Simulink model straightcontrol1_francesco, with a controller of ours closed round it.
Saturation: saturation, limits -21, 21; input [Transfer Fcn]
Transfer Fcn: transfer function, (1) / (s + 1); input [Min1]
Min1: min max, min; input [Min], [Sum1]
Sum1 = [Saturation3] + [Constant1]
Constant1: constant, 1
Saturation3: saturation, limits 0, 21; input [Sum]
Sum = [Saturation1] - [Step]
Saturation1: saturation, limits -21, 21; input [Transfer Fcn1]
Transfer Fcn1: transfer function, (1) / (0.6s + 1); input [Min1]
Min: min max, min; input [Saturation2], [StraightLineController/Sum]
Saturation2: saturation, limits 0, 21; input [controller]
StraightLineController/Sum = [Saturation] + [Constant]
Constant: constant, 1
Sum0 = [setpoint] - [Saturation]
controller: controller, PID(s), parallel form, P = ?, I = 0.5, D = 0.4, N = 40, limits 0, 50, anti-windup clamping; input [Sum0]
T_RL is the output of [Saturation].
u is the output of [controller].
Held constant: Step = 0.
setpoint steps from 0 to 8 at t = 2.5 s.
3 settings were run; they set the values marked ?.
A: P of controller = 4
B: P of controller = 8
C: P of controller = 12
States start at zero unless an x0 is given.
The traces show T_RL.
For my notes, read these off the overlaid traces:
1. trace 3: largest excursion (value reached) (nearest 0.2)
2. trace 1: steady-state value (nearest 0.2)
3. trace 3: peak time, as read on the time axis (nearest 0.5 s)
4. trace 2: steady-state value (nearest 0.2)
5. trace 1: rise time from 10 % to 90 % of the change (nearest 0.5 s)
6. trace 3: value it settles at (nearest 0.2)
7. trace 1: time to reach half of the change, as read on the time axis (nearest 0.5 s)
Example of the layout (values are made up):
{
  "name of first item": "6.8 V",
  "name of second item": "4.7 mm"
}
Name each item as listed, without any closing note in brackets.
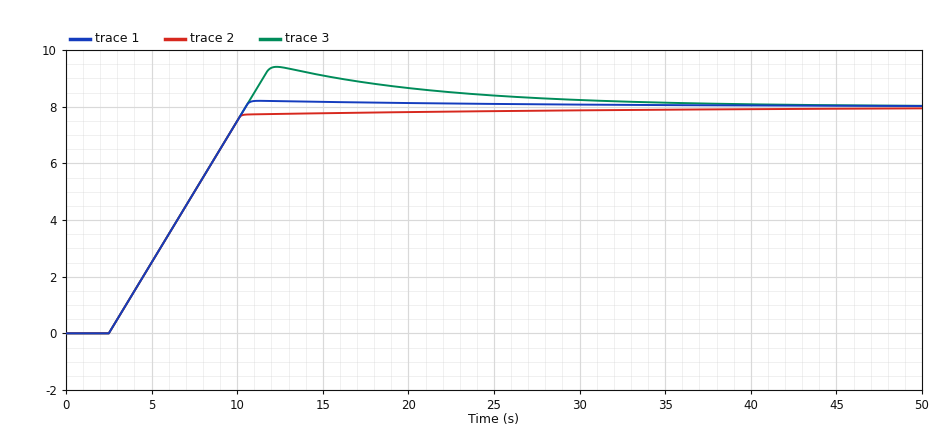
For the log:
{
  "trace 3: largest excursion (value reached)": "9.4",
  "trace 1: steady-state value": "8.0",
  "trace 3: peak time, as read on the time axis": "12.5 s",
  "trace 2: steady-state value": "8.0",
  "trace 1: rise time from 10 % to 90 % of the change": "6.5 s",
  "trace 3: value it settles at": "8.0",
  "trace 1: time to reach half of the change, as read on the time axis": "6.5 s"
}
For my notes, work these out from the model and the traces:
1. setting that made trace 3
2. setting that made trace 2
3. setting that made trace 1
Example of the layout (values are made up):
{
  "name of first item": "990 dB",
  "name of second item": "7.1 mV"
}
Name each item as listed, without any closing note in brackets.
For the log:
{
  "setting that made trace 3": "A",
  "setting that made trace 2": "C",
  "setting that made trace 1": "B"
}
